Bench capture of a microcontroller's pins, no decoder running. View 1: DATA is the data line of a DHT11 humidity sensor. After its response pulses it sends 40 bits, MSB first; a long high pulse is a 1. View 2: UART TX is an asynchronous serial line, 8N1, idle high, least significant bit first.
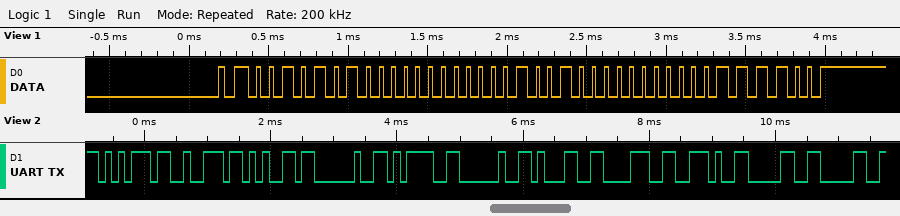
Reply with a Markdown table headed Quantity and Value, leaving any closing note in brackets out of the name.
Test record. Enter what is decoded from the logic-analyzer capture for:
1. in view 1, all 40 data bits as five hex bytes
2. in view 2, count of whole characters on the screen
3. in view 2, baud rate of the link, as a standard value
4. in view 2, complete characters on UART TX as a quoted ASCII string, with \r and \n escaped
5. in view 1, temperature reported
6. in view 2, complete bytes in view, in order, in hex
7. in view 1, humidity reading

| Quantity | Value |
|---|---|
| in view 1, all 40 data bits as five hex bytes | 2A 00 12 00 3C |
| in view 2, count of whole characters on the screen | 11 |
| in view 2, baud rate of the link, as a standard value | 9600 baud |
| in view 2, complete characters on UART TX as a quoted ASCII string, with \r and \n escaped | "ure = 18.00" |
| in view 1, temperature reported | 18.0 °C |
| in view 2, complete bytes in view, in order, in hex | 0x75 0x72 0x65 0x20 0x3D 0x20 0x31 0x38 0x2E 0x30 0x30 |
| in view 1, humidity reading | 42 % |
